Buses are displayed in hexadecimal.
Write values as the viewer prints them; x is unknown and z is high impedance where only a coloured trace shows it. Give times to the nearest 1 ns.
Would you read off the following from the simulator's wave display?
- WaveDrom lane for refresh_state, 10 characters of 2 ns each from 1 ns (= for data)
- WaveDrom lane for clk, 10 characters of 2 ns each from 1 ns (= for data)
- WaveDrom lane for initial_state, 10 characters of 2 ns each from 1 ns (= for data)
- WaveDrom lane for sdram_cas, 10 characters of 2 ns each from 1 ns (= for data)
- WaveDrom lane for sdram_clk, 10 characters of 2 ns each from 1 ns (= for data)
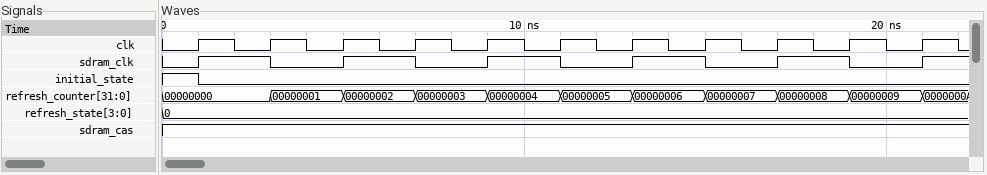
{name: 'refresh_state', wave: '=.........', data: '0'}
{name: 'clk', wave: 'p.........'}
{name: 'initial_state', wave: '0.........'}
{name: 'sdram_cas', wave: '1.........'}
{name: 'sdram_clk', wave: '1010101010'}
